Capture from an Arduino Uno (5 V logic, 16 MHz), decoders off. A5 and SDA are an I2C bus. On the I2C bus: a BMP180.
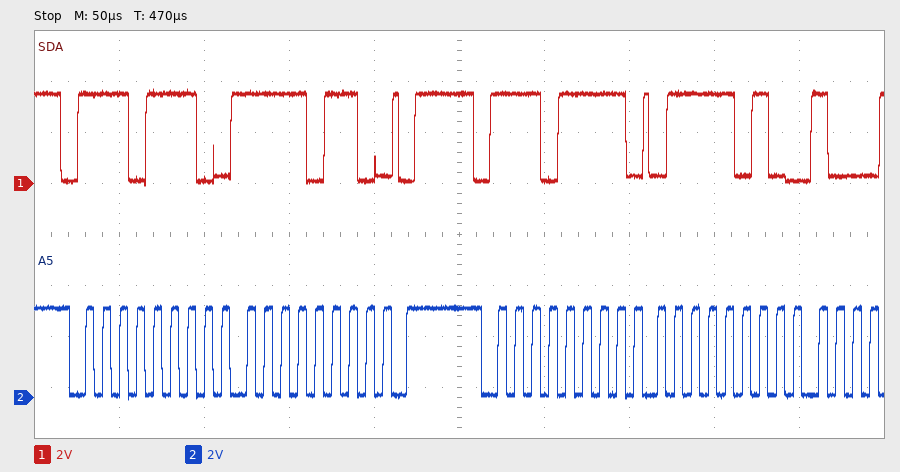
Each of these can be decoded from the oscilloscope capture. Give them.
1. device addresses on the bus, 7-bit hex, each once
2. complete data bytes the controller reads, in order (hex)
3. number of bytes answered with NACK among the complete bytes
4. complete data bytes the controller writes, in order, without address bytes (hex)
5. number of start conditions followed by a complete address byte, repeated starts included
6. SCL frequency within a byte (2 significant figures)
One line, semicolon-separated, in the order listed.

0x77; 7A; 0; F6; 2; 100 kHz
